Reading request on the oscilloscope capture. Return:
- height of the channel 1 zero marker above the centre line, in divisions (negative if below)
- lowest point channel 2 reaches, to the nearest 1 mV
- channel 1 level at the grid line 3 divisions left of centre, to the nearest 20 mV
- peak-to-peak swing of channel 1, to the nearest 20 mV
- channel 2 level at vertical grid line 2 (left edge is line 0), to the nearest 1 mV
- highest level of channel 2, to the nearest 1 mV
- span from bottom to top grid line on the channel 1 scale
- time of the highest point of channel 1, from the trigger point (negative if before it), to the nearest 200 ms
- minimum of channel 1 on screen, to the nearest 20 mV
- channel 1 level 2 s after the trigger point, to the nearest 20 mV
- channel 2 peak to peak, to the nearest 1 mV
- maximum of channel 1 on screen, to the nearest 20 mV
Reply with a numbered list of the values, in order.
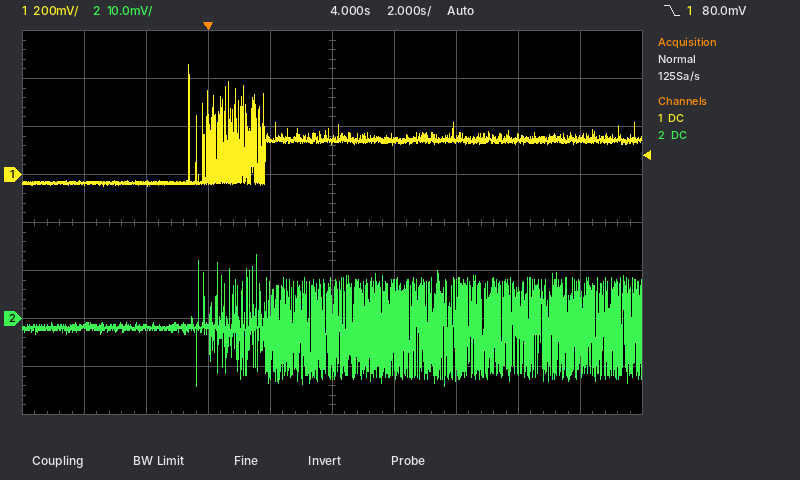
1. +1.0 div
2. -14 mV
3. -40 mV
4. 500 mV
5. -2 mV
6. 13 mV
7. 1.6 V
8. -600 ms
9. -40 mV
10. 160 mV
11. 27 mV
12. 460 mV
